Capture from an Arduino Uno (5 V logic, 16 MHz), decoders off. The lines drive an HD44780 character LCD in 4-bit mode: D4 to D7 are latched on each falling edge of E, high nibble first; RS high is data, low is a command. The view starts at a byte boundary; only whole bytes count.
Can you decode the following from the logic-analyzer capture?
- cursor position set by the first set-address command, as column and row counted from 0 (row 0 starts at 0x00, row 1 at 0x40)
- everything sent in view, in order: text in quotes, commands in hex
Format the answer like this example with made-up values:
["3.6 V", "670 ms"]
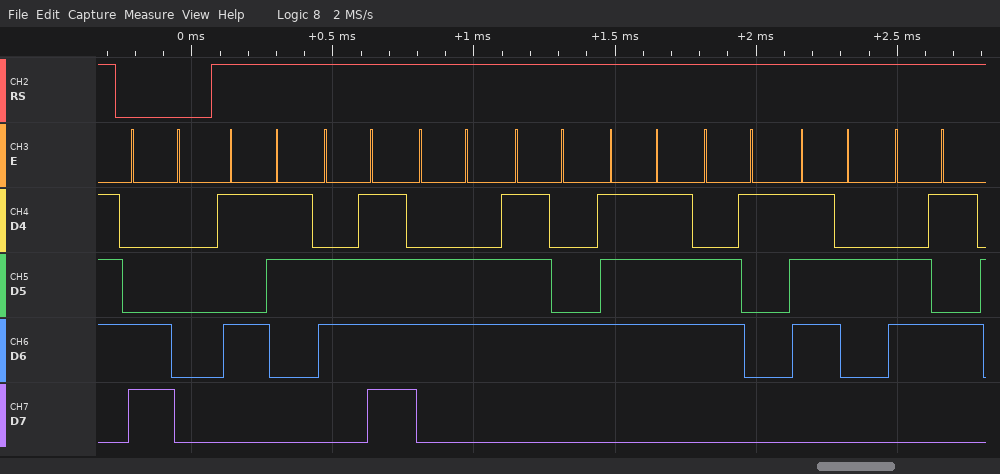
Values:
["column 0, row 1", "0xC0 \"Software\""]
